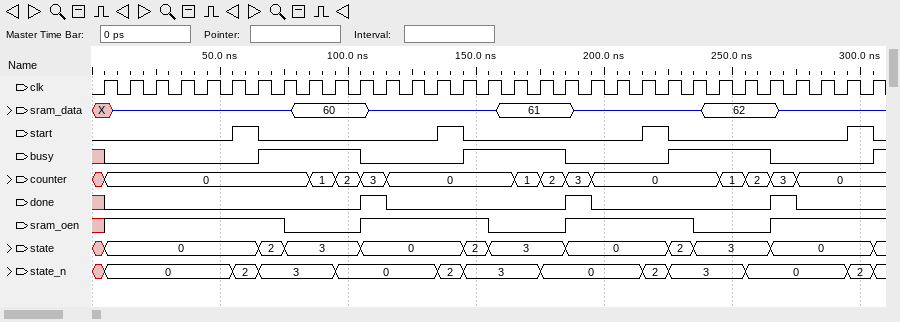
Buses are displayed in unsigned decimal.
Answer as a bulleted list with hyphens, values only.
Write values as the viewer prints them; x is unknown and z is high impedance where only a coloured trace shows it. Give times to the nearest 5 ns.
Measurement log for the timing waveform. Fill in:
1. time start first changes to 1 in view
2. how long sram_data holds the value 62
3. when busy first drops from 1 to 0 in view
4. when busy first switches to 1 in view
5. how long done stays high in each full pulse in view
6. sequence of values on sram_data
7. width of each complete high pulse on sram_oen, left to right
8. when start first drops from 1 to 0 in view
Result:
- 55 ns
- 30 ns
- 105 ns
- 65 ns
- 10 ns, 10 ns, 10 ns
- X, z, 60, z, 61, z, 62, z
- 50 ns, 50 ns
- 65 ns
